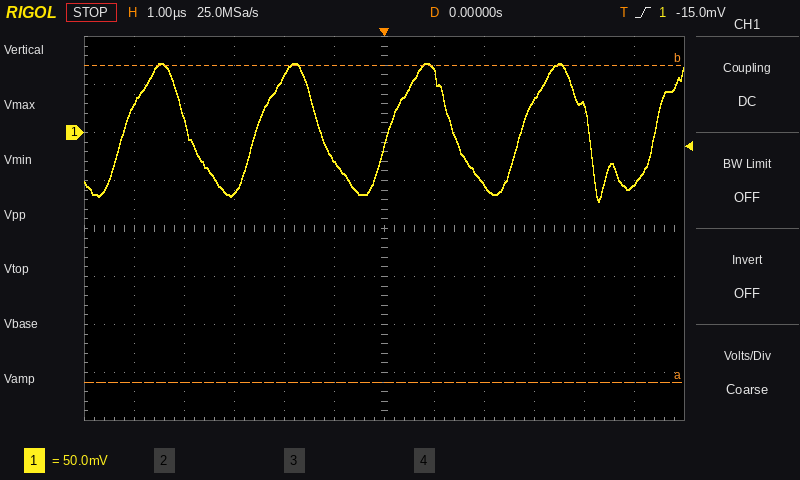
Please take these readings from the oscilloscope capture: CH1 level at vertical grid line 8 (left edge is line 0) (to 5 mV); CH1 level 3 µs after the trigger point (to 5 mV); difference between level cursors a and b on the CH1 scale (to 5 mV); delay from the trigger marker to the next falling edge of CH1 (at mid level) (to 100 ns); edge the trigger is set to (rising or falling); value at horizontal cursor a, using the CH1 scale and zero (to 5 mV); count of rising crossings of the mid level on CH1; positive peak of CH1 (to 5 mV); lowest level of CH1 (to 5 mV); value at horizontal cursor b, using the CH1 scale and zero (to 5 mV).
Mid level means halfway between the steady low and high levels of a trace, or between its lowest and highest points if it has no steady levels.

-55 mV
35 mV
330 mV
1.4 µs
rising
-260 mV
5
70 mV
-70 mV
70 mV
